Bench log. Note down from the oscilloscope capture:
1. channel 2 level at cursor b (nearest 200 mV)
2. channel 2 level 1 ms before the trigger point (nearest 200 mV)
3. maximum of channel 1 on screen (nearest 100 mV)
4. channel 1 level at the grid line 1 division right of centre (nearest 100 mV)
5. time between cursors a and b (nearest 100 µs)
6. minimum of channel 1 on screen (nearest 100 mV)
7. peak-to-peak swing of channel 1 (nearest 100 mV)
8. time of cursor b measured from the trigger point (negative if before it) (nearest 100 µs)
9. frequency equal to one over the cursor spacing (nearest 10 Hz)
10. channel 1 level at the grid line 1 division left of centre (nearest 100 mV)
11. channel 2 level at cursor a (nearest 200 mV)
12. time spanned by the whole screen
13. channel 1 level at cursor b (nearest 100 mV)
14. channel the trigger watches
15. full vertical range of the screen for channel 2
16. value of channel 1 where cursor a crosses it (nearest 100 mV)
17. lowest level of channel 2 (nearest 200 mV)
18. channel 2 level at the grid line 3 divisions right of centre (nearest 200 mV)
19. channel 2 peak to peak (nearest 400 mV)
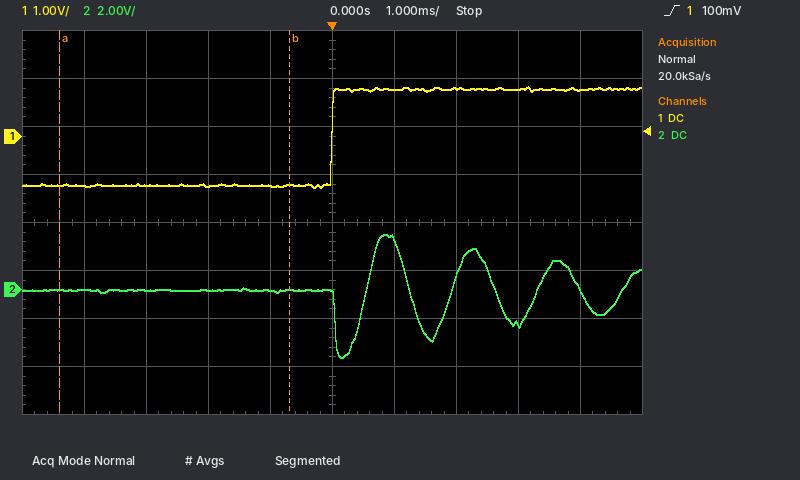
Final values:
0.0 V
0.0 V
1.0 V
1.0 V
3.7 ms
-1.1 V
2.1 V
-700 µs
270 Hz
-1.0 V
0.0 V
10 ms
-1.0 V
channel 1
16 V
-1.0 V
-2.8 V
-1.4 V
5.2 V
